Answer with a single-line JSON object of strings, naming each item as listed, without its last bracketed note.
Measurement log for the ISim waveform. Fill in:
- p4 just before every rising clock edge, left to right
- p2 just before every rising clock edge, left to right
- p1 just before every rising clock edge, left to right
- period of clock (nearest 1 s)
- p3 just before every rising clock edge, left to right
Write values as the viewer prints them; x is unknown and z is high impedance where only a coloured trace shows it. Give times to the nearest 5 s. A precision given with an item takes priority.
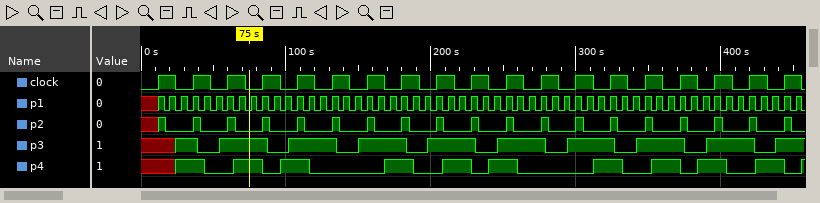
{"p4 just before every rising clock edge, left to right": "x 1 0 1 1 0 0 1 0 1 1 0 0 1 0 1 1 0 1", "p2 just before every rising clock edge, left to right": "x 0 0 0 0 0 0 0 0 0 0 0 0 0 0 0 0 0 0", "p1 just before every rising clock edge, left to right": "x 0 0 0 0 0 0 0 0 0 0 0 0 0 0 0 0 0 0", "period of clock": "24 s", "p3 just before every rising clock edge, left to right": "x 1 1 1 1 1 1 1 1 1 1 1 1 1 1 1 1 1 1"}
